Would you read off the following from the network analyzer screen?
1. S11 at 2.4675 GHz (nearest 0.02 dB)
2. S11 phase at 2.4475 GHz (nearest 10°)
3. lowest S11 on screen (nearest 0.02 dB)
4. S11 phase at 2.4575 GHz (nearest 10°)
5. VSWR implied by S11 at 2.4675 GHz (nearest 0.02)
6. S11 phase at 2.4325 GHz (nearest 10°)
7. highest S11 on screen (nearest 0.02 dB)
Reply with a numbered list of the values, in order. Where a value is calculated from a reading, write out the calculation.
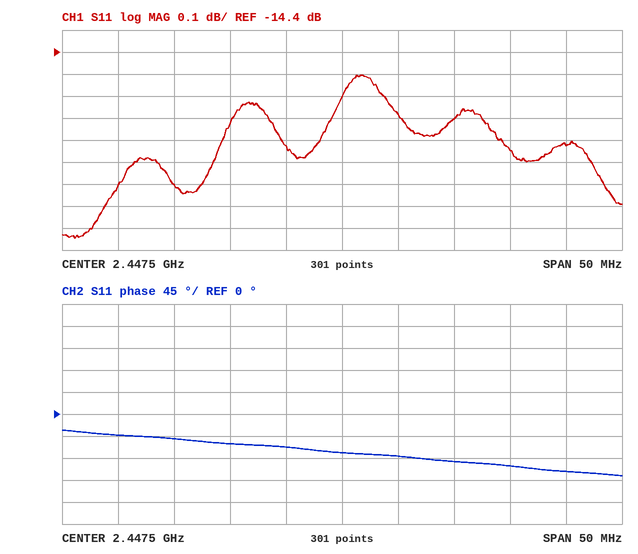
1. -14.82 dB
2. -80°
3. -15.24 dB
4. -100°
5. |Γ| = 10^(-14.82/20) = 0.1816; VSWR = (1 + 0.1816)/(1 − 0.1816) ≈ 1.44
6. -50°
7. -14.50 dB
